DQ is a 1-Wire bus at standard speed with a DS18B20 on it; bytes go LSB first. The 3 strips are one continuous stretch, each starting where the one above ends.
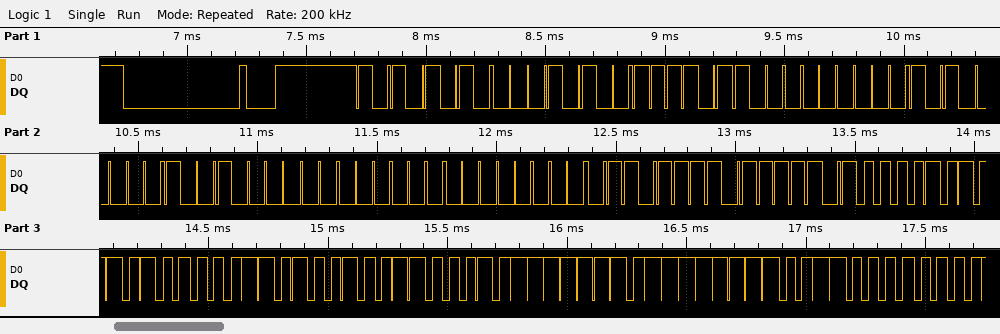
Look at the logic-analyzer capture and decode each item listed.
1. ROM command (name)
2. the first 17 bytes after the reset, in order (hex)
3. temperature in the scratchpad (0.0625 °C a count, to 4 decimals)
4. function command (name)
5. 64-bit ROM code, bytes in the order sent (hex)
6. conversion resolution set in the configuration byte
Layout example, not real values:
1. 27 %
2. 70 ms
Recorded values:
1. Match ROM
2. 55 28 6F 00 05 09 00 00 F6 BE 50 05 4B 46 7F FF 0C
3. 85.0000 °C
4. Read Scratchpad
5. 28 6F 00 05 09 00 00 F6
6. 12 bits
